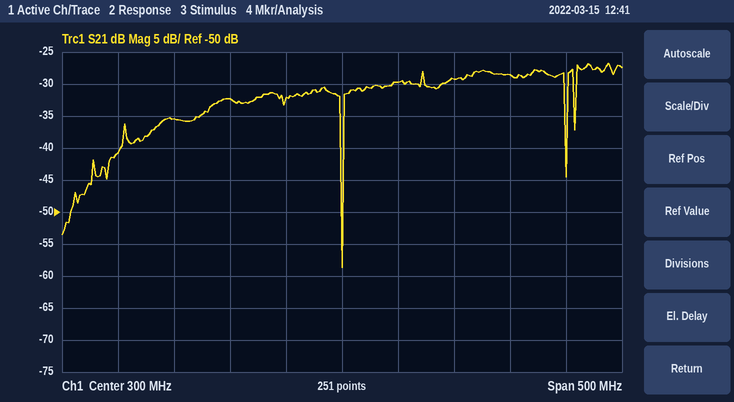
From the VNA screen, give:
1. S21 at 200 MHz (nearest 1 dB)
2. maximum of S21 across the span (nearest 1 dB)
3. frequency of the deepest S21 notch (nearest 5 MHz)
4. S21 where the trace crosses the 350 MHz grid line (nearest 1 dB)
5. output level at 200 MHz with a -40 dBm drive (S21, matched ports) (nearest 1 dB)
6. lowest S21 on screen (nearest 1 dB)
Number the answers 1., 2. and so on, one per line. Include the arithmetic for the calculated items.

1. -32 dB
2. -27 dB
3. 300 MHz
4. -30 dB
5. -40 dBm + (-32 dB) = -72 dBm
6. -59 dB
